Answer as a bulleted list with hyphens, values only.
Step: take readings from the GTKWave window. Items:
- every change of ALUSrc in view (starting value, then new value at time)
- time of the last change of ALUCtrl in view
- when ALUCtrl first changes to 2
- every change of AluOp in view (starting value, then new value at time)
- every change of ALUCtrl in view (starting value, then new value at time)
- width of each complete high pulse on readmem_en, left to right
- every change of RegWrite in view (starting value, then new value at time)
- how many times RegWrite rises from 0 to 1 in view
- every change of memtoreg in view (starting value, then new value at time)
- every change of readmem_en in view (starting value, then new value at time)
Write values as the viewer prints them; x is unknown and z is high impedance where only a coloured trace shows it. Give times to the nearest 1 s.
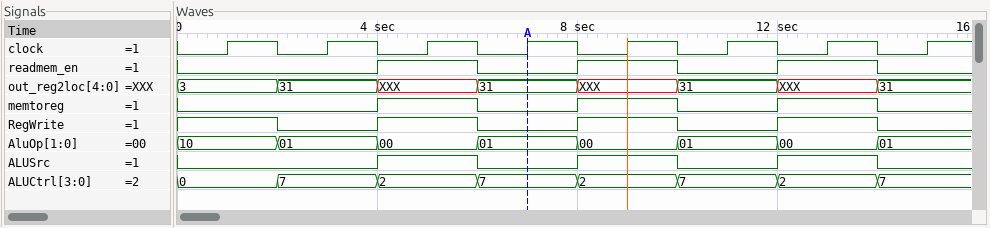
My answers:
- 0, 1 at 4 s, 0 at 6 s, 1 at 8 s, 0 at 10 s, 1 at 12 s, 0 at 14 s
- 14 s
- 4 s
- 10, 01 at 2 s, 00 at 4 s, 01 at 6 s, 00 at 8 s, 01 at 10 s, 00 at 12 s, 01 at 14 s
- 0, 7 at 2 s, 2 at 4 s, 7 at 6 s, 2 at 8 s, 7 at 10 s, 2 at 12 s, 7 at 14 s
- 2 s, 2 s, 2 s
- 1, 0 at 2 s, 1 at 4 s, 0 at 6 s, 1 at 8 s, 0 at 10 s, 1 at 12 s, 0 at 14 s
- 3
- 0, 1 at 4 s, 0 at 6 s, 1 at 8 s, 0 at 10 s, 1 at 12 s, 0 at 14 s
- 0, 1 at 4 s, 0 at 6 s, 1 at 8 s, 0 at 10 s, 1 at 12 s, 0 at 14 s
